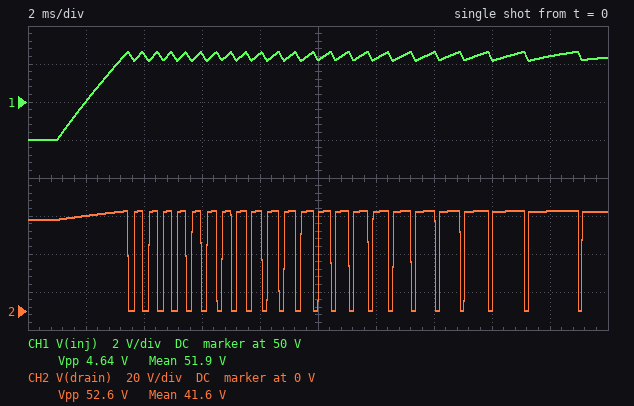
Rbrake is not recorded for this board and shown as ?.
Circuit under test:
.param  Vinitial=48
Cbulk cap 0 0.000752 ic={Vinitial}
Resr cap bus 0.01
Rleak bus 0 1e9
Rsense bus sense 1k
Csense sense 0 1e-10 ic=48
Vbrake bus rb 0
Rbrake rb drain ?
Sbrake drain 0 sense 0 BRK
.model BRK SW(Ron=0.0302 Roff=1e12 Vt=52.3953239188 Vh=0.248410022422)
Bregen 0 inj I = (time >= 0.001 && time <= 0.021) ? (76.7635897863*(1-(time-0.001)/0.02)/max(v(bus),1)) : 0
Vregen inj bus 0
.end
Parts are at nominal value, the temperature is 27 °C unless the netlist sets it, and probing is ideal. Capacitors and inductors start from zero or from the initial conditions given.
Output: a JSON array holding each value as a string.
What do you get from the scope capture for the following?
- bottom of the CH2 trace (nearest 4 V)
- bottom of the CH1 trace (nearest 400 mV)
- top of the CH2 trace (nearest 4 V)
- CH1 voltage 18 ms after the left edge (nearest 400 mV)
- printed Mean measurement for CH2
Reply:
["0 V", "48.0 V", "52 V", "52.4 V", "41.6 V"]
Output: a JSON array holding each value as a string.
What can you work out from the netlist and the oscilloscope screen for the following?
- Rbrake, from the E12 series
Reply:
["18 Ω"]
